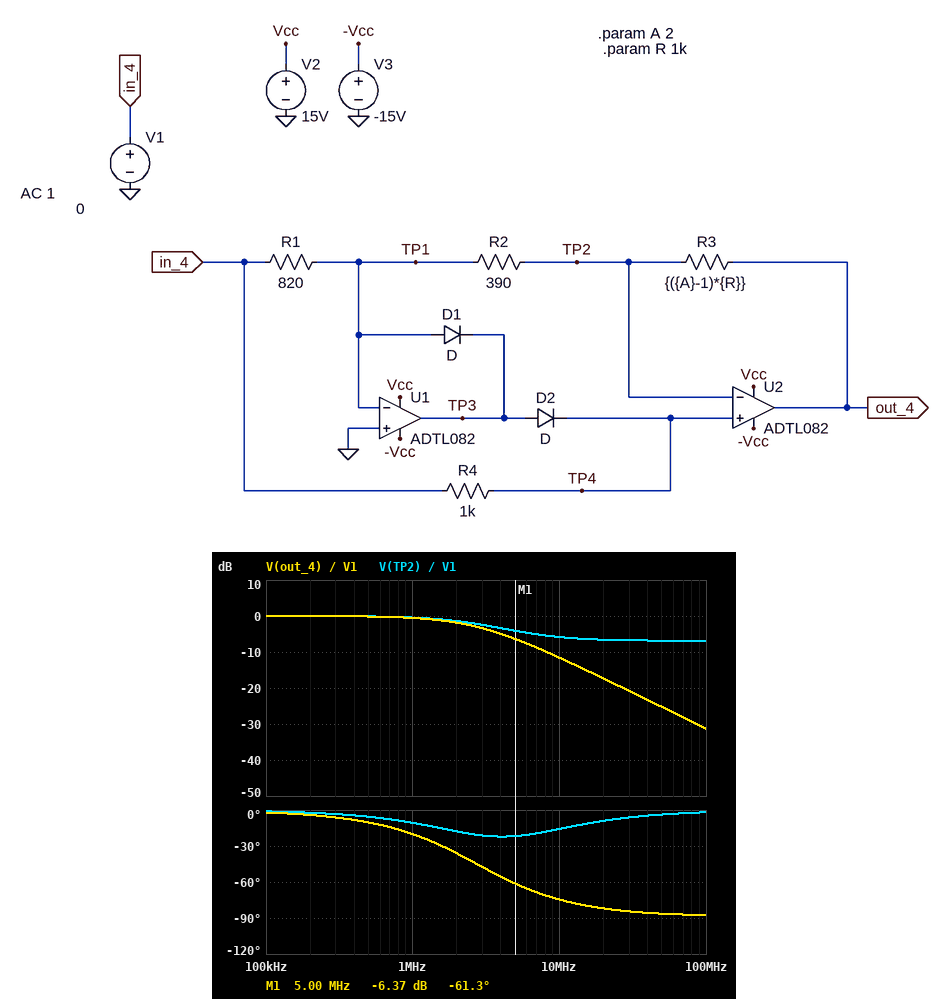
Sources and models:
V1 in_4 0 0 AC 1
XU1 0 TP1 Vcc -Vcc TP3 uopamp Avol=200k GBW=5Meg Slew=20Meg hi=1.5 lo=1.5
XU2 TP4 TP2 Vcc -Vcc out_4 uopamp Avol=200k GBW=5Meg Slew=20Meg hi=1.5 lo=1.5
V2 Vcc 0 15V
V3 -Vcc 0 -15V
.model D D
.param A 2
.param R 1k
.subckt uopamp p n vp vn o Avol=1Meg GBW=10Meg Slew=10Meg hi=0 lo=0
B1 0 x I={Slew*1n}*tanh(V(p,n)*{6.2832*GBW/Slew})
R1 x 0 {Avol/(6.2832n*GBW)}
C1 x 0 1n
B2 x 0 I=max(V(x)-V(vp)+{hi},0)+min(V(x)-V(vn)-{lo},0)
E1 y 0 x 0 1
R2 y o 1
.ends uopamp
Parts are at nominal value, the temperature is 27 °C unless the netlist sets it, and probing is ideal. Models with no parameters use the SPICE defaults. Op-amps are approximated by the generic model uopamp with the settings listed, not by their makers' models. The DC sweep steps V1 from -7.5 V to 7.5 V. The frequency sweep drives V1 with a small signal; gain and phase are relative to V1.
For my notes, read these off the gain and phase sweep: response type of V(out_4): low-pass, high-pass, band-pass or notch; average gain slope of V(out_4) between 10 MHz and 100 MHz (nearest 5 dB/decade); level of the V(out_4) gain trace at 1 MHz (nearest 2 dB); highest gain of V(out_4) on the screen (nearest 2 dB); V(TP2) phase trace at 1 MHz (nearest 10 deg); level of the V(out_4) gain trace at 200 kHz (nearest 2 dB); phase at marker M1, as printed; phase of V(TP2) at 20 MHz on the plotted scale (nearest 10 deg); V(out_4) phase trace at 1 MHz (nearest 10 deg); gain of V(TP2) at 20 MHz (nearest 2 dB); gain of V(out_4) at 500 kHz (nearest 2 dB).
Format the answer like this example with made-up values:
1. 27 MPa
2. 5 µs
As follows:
1. low-pass
2. -20 dB/decade
3. 0 dB
4. 0 dB
5. -10 deg
6. 0 dB
7. -61.3 deg
8. -10 deg
9. -20 deg
10. -6 dB
11. 0 dB
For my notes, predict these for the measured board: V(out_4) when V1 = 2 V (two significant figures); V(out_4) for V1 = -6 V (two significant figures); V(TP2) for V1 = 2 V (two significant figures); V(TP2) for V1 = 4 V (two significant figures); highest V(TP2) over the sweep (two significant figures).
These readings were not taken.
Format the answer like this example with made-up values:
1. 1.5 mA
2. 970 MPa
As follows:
1. 7.1 V
2. 10 V
3. 2.0 V
4. 3.8 V
5. 3.8 V
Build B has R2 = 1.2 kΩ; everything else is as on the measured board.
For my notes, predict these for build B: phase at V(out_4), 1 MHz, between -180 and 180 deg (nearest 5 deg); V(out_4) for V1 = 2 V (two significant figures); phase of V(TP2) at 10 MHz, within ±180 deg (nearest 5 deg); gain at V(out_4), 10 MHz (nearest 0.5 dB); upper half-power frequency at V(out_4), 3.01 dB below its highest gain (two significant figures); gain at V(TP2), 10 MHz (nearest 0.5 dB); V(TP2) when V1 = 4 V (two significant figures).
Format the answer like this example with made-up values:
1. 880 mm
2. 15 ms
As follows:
1. -15 deg
2. 3.7 V
3. -25 deg
4. -10.0 dB
5. 3.3 MHz
6. -7.0 dB
7. 4.0 V
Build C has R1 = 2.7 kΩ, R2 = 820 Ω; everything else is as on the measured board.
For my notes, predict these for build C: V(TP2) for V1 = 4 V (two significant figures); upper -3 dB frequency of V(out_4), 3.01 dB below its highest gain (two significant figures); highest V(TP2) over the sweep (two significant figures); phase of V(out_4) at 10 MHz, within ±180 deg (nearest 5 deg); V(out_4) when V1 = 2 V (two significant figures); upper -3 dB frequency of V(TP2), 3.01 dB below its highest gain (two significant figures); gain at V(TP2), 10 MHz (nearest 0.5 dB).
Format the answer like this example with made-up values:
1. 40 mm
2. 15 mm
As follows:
1. 4.0 V
2. 3.9 MHz
3. 6.1 V
4. -70 deg
5. 4.4 V
6. 4.1 MHz
7. -7.5 dB
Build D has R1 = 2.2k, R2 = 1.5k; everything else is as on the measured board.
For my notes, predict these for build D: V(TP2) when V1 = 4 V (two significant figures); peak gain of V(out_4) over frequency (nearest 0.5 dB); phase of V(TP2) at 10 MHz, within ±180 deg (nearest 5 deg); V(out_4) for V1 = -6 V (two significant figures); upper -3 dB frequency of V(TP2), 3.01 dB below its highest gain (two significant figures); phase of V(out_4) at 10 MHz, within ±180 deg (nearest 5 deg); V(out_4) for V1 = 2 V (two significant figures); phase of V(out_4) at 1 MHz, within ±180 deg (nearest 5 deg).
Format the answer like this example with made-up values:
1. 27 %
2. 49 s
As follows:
1. 4.0 V
2. 0 dB
3. -40 deg
4. 6.8 V
5. 4.1 MHz
6. -70 deg
7. 3.3 V
8. -15 deg
